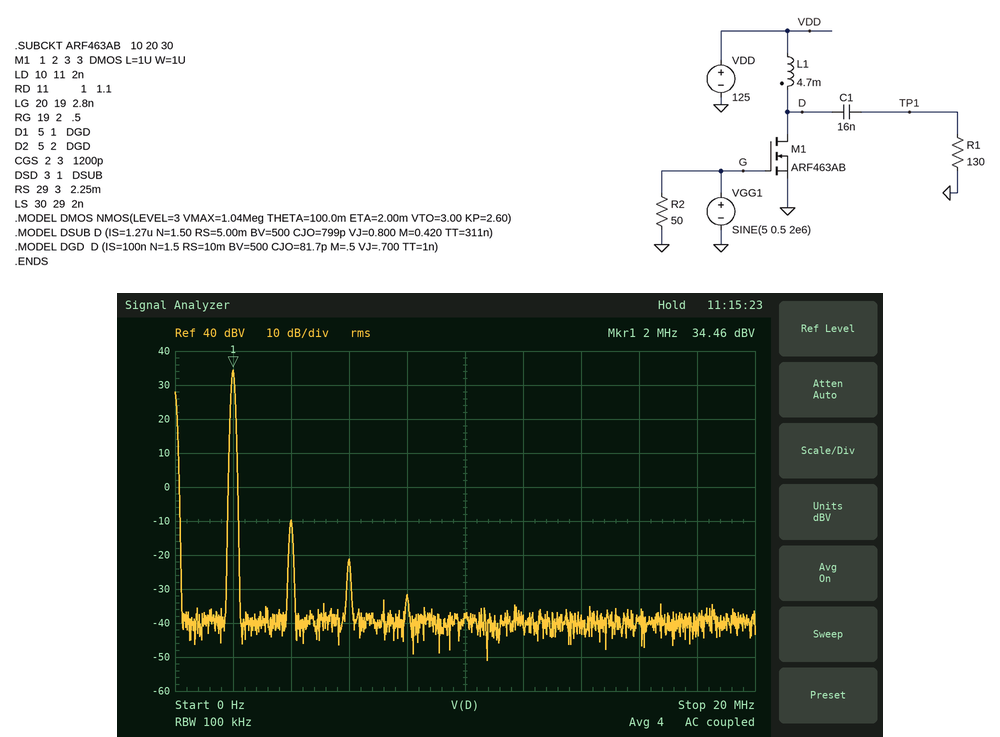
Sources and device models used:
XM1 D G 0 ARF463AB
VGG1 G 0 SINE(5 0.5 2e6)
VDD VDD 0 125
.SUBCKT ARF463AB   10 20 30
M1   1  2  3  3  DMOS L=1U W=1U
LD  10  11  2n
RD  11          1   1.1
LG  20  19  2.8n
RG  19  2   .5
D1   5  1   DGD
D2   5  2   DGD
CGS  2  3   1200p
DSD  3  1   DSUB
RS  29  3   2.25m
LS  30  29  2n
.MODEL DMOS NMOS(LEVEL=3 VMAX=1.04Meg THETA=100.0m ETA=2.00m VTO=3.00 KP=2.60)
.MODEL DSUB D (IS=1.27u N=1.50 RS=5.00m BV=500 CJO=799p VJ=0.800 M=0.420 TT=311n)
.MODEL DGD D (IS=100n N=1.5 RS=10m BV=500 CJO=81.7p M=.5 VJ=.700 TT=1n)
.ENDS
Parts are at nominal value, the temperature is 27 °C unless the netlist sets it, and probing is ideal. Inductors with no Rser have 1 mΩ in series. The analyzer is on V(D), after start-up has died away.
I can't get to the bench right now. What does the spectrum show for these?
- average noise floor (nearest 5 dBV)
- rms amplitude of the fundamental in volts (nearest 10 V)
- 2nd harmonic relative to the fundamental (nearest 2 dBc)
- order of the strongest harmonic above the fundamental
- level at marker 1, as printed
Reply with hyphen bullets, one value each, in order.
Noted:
- -40 dBV
- 50 V
- -44 dBc
- 2
- 34.46 dBV
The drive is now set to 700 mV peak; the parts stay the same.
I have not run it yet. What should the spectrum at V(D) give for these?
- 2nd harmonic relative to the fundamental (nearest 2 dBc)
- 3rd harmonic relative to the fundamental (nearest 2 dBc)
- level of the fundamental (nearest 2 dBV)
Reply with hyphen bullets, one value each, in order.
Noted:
- -40 dBc
- -46 dBc
- 38 dBV
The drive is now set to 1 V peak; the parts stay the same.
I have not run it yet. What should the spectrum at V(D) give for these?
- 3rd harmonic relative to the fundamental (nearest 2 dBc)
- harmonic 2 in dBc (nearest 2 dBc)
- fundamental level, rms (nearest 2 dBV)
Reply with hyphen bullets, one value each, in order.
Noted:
- -26 dBc
- -24 dBc
- 40 dBV
